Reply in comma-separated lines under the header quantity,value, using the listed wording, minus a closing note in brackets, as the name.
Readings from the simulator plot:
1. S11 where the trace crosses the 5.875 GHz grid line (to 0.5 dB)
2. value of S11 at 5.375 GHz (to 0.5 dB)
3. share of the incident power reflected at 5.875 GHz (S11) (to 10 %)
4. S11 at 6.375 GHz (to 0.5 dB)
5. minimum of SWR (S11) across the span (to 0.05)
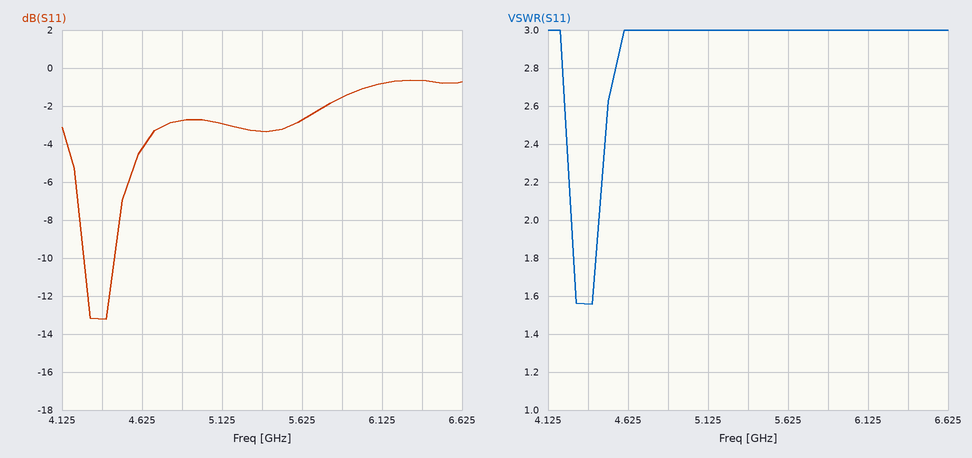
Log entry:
quantity,value
S11 where the trace crosses the 5.875 GHz grid line,-1.5 dB
value of S11 at 5.375 GHz,-3.5 dB
share of the incident power reflected at 5.875 GHz (S11),70 %
S11 at 6.375 GHz,-0.5 dB
minimum of SWR (S11) across the span,1.55
